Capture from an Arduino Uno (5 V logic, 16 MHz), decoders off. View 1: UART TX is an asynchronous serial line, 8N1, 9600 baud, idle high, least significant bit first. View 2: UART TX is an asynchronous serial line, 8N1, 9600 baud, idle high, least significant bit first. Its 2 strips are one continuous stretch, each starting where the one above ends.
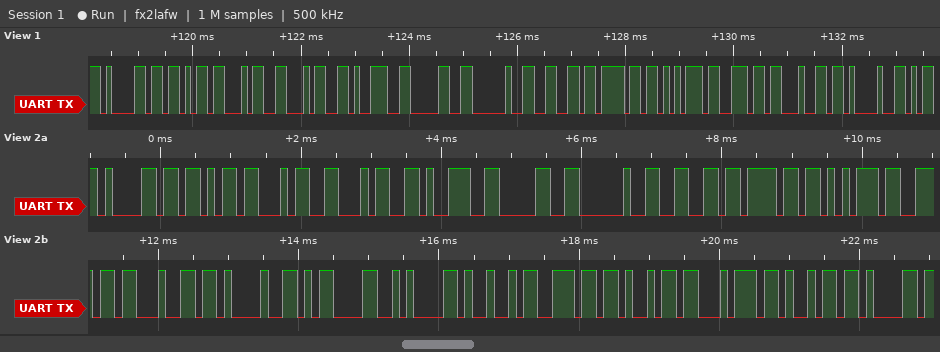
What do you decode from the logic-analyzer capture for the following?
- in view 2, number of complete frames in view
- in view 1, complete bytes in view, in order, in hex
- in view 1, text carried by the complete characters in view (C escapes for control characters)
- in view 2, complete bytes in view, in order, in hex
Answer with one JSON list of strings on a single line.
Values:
["21", "0x61 0x6B 0x34 0x34 0x39 0x30 0x20 0x66 0x6F 0x75 0x6E 0x64 0x21", "\"ak4490 found!\"", "0x61 0x6B 0x34 0x34 0x39 0x30 0x20 0x66 0x6F 0x75 0x6E 0x64 0x21 0x0D 0x0A 0x49 0x6E 0x69 0x74 0x69 0x61"]
